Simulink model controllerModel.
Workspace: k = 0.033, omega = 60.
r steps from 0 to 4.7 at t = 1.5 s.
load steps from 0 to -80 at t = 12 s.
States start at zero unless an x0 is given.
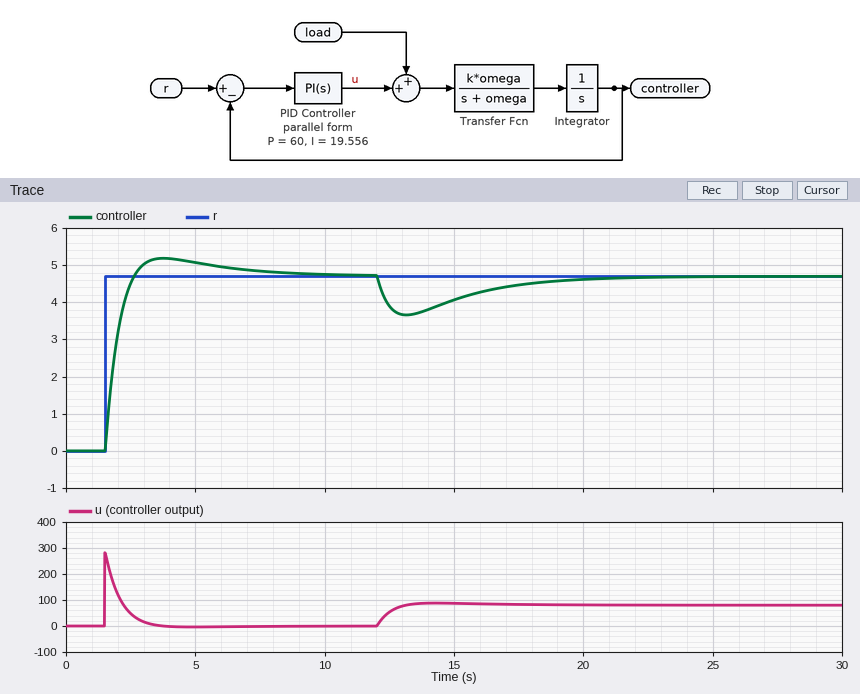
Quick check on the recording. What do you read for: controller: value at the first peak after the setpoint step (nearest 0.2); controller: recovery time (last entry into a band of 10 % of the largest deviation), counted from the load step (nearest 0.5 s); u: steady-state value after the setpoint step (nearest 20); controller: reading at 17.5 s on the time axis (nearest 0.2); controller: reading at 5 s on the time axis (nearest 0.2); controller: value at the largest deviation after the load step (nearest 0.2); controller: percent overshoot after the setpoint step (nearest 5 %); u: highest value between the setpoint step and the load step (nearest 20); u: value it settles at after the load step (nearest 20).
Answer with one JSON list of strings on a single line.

["5.2", "7.5 s", "0", "4.4", "5.0", "3.6", "10 %", "280", "80"]
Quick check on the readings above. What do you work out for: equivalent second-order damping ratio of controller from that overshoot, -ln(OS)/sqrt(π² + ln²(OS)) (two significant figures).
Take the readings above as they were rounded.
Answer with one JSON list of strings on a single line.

["0.59"]
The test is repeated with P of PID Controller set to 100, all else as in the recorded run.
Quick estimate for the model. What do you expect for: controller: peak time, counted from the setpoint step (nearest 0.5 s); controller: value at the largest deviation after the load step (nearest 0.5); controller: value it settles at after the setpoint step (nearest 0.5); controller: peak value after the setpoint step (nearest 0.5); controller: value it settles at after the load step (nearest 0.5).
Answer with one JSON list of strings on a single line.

["2.0 s", "4.0", "4.5", "5.0", "4.5"]
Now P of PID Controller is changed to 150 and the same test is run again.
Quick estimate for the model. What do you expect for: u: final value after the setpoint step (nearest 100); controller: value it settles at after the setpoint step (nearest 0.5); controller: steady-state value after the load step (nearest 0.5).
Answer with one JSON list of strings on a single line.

["0", "4.5", "4.5"]
